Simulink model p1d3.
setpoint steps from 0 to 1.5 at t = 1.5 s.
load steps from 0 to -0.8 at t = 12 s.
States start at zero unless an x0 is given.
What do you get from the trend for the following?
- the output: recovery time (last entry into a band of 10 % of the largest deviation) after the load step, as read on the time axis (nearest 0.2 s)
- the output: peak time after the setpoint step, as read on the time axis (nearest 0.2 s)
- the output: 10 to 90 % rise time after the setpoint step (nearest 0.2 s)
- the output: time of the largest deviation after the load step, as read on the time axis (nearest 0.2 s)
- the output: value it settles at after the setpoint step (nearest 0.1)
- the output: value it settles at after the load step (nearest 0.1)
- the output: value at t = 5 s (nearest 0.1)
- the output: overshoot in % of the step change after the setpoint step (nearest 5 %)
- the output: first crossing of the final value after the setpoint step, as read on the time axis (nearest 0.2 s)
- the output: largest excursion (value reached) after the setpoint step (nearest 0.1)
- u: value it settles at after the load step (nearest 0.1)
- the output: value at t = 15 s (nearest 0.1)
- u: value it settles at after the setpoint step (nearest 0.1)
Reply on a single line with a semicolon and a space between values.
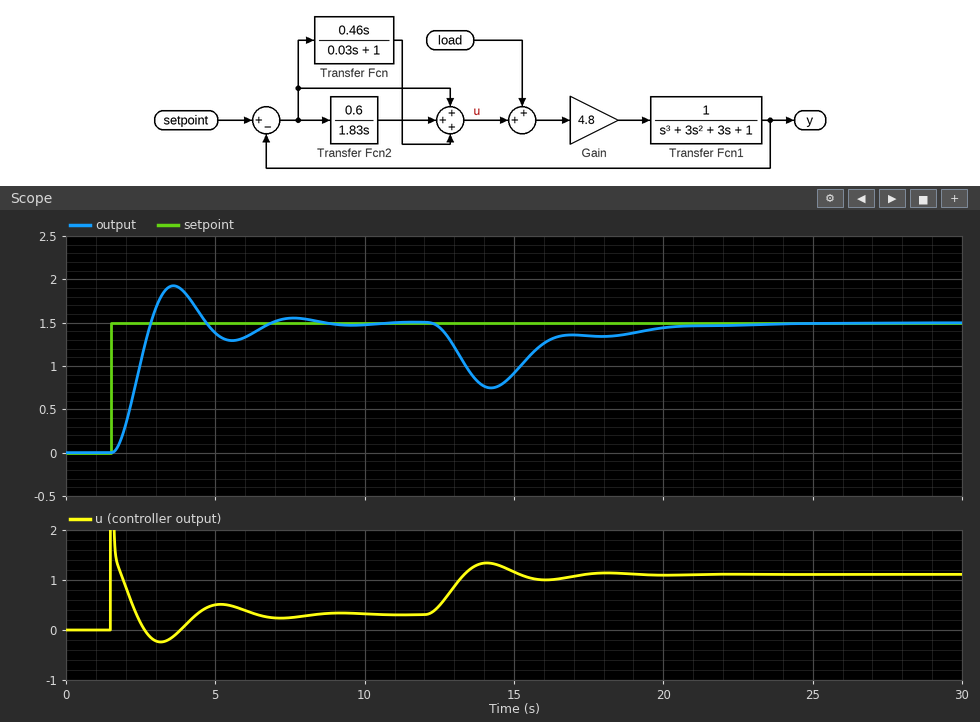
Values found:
19.6 s; 3.6 s; 0.8 s; 14.2 s; 1.5; 1.5; 1.4; 30 %; 2.8 s; 1.9; 1.1; 0.9; 0.3
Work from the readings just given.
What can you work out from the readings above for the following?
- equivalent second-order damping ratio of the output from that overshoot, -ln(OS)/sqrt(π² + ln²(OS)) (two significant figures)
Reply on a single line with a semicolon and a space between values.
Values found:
0.36
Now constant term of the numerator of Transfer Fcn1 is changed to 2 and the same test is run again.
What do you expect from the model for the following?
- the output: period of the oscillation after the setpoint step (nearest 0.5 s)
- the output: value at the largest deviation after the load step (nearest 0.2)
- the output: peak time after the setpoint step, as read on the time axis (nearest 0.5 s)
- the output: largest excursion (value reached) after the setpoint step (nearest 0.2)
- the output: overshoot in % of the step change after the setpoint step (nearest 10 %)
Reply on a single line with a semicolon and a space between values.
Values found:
3.0 s; 0.6; 3.0 s; 2.2; 50 %
